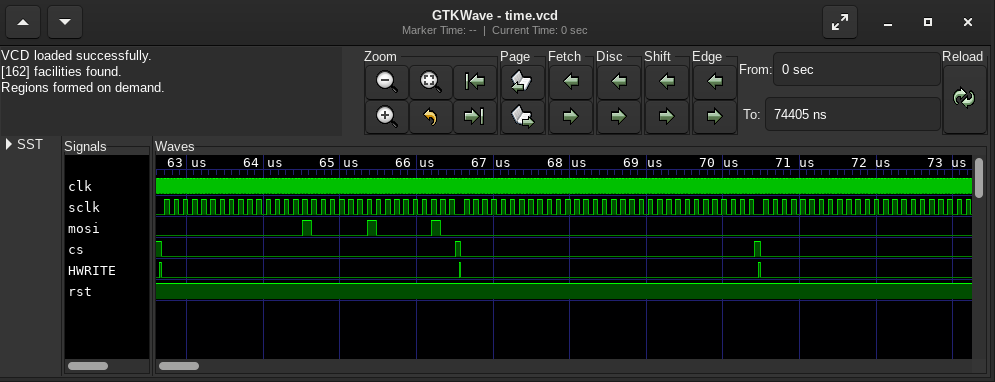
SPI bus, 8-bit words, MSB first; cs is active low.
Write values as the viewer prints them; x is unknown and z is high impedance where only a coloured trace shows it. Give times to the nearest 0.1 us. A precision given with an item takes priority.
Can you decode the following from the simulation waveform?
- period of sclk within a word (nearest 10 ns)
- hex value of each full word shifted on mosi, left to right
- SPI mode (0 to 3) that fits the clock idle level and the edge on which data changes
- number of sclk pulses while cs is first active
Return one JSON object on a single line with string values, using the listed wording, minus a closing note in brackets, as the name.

{"period of sclk within a word": "120 ns", "hex value of each full word shifted on mosi, left to right": "00, 01, 02, 04, 00, 00, 00, 00, 00, 00", "SPI mode (0 to 3) that fits the clock idle level and the edge on which data changes": "1", "number of sclk pulses while cs is first active": "32"}
